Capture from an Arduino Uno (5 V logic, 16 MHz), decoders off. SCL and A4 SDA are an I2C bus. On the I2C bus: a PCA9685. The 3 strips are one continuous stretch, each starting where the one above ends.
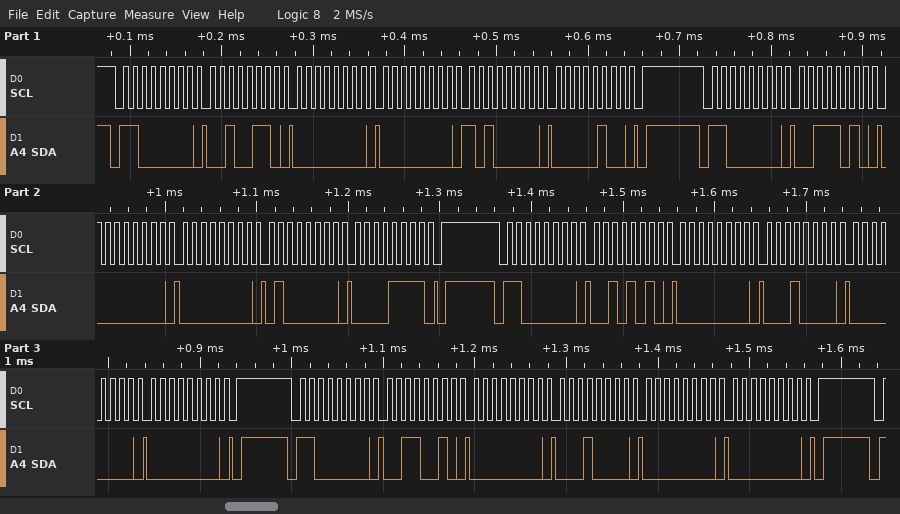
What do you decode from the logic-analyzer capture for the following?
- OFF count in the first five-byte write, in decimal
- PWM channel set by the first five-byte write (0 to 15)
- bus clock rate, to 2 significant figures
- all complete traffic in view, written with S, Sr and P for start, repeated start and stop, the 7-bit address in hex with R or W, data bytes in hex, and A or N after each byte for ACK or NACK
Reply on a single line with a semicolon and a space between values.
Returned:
1184; 8; 100 kHz; S 60W A 26 A 00 A 00 A A0 A 04 A P S 60W A 3A A 00 A 00 A 40 A 0F A P S 60W A 2A A 00 A 10 A 00 A 00 A P S 60W A 32 A 00 A 10 A 00 A 00 A P
